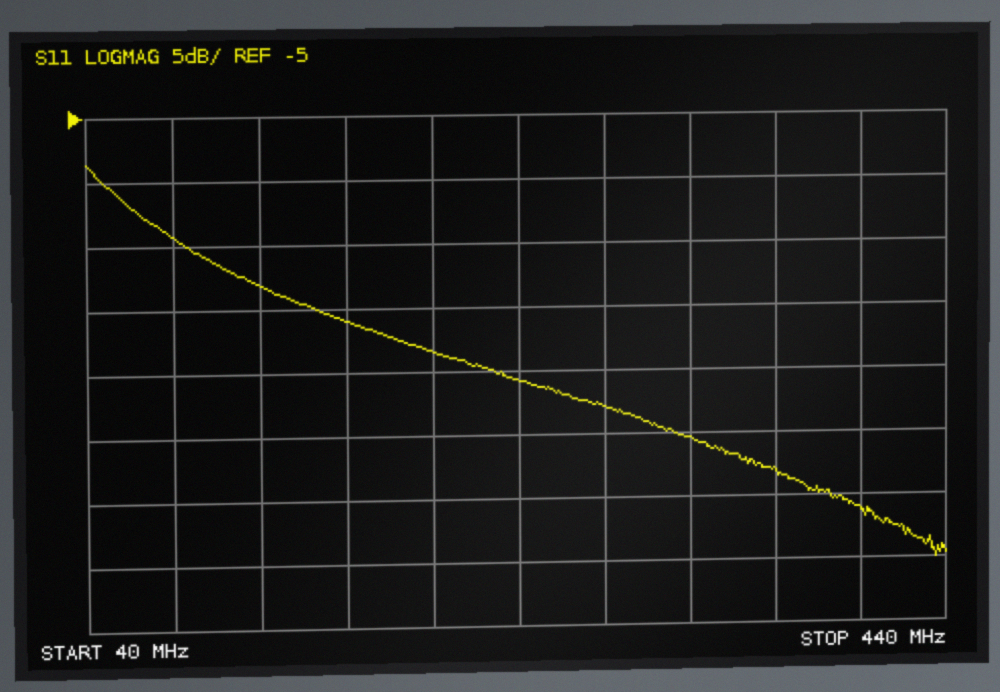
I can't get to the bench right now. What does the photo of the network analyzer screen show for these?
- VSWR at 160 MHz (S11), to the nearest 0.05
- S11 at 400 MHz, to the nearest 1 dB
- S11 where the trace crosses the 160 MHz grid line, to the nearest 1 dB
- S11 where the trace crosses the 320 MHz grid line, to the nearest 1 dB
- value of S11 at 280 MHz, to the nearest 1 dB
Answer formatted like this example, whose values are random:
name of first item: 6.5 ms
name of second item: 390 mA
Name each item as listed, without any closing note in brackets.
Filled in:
VSWR at 160 MHz (S11), to the nearest 0.05: 1.20
S11 at 400 MHz, to the nearest 1 dB: -36 dB
S11 where the trace crosses the 160 MHz grid line, to the nearest 1 dB: -21 dB
S11 where the trace crosses the 320 MHz grid line, to the nearest 1 dB: -30 dB
value of S11 at 280 MHz, to the nearest 1 dB: -28 dB
